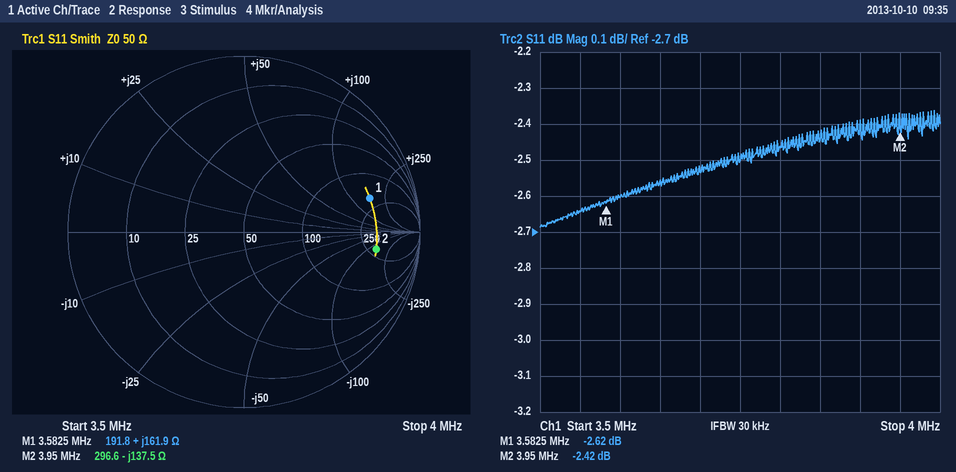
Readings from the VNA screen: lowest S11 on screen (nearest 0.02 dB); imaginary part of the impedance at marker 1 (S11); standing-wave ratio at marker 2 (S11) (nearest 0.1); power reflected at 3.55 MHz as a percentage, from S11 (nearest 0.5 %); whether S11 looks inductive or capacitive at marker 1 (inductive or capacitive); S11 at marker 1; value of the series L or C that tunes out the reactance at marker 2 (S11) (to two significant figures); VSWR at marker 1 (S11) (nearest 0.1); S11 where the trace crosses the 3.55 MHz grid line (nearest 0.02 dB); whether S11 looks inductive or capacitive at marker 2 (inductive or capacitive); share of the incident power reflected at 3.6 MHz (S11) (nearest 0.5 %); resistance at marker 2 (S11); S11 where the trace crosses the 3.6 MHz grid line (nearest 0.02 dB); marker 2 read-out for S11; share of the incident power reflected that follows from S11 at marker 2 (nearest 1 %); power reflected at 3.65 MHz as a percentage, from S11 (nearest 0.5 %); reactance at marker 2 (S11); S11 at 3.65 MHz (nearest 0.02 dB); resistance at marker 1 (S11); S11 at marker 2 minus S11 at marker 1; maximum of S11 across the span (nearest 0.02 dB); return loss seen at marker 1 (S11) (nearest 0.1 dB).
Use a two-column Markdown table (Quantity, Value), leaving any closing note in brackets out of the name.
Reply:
| Quantity | Value |
|---|---|
| lowest S11 on screen | -2.68 dB |
| imaginary part of the impedance at marker 1 | +161.9 Ω |
| standing-wave ratio at marker 2 (S11) | 7.2 |
| power reflected at 3.55 MHz as a percentage, from S11 | 54.5 % |
| whether S11 looks inductive or capacitive at marker 1 | inductive |
| S11 at marker 1 | -2.62 dB |
| value of the series L or C that tunes out the reactance at marker 2 (S11) | 5.5 µH |
| VSWR at marker 1 (S11) | 6.7 |
| S11 where the trace crosses the 3.55 MHz grid line | -2.64 dB |
| whether S11 looks inductive or capacitive at marker 2 | capacitive |
| share of the incident power reflected at 3.6 MHz (S11) | 55.0 % |
| resistance at marker 2 | 296.6 Ω |
| S11 where the trace crosses the 3.6 MHz grid line | -2.60 dB |
| marker 2 read-out for S11 | -2.42 dB |
| share of the incident power reflected that follows from S11 at marker 2 | 57 % |
| power reflected at 3.65 MHz as a percentage, from S11 | 55.5 % |
| reactance at marker 2 | -137.5 Ω |
| S11 at 3.65 MHz | -2.56 dB |
| resistance at marker 1 | 191.8 Ω |
| S11 at marker 2 minus S11 at marker 1 | 0.20 dB |
| maximum of S11 across the span | -2.36 dB |
| return loss seen at marker 1 (S11) | 2.6 dB |
